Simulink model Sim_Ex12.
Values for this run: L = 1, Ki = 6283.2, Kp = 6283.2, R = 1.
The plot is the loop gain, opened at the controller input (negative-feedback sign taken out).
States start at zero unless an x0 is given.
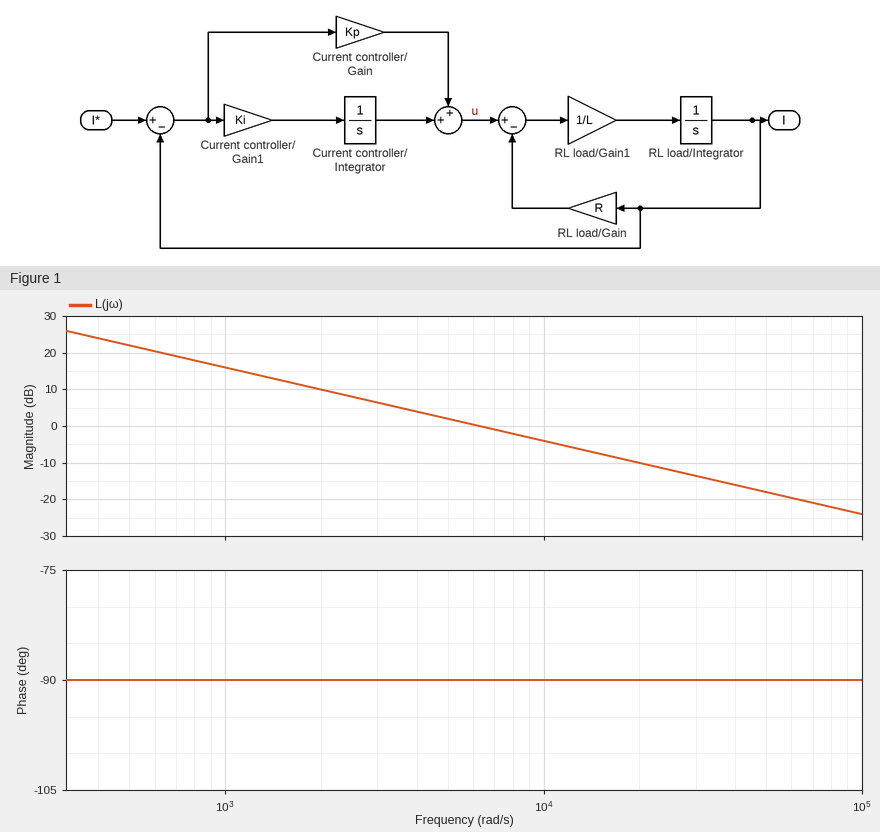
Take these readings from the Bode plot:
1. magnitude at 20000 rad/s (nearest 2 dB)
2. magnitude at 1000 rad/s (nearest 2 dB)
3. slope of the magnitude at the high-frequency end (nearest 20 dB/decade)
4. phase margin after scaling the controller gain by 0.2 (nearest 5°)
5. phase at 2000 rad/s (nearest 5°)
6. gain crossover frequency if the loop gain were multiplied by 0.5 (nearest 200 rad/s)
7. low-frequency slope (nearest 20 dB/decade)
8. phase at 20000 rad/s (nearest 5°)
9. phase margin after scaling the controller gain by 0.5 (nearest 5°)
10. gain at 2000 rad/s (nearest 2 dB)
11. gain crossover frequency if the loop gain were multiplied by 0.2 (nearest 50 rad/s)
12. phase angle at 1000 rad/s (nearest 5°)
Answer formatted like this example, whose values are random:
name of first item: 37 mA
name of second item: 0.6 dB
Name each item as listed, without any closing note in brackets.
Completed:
magnitude at 20000 rad/s: -10 dB
magnitude at 1000 rad/s: 16 dB
slope of the magnitude at the high-frequency end: -20 dB/decade
phase margin after scaling the controller gain by 0.2: 90°
phase at 2000 rad/s: -90°
gain crossover frequency if the loop gain were multiplied by 0.5: 3200 rad/s
low-frequency slope: -20 dB/decade
phase at 20000 rad/s: -90°
phase margin after scaling the controller gain by 0.5: 90°
gain at 2000 rad/s: 10 dB
gain crossover frequency if the loop gain were multiplied by 0.2: 1250 rad/s
phase angle at 1000 rad/s: -90°
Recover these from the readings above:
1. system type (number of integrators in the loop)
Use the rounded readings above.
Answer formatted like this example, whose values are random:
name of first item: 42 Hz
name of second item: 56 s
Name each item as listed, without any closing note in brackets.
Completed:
system type: 1
